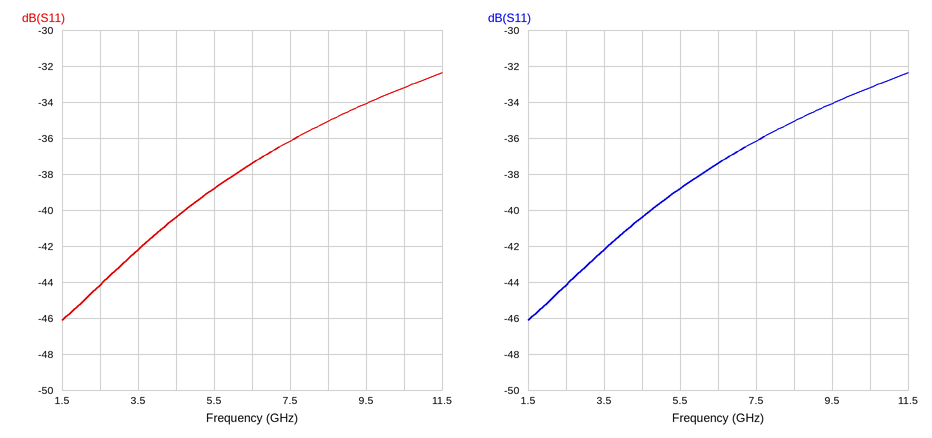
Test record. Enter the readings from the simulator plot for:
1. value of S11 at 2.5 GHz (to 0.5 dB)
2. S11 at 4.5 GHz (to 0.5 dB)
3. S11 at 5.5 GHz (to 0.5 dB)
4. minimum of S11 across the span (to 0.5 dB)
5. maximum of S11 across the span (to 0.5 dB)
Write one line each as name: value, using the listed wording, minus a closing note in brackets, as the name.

value of S11 at 2.5 GHz: -44.0 dB
S11 at 4.5 GHz: -40.5 dB
S11 at 5.5 GHz: -39.0 dB
minimum of S11 across the span: -46.0 dB
maximum of S11 across the span: -32.5 dB
